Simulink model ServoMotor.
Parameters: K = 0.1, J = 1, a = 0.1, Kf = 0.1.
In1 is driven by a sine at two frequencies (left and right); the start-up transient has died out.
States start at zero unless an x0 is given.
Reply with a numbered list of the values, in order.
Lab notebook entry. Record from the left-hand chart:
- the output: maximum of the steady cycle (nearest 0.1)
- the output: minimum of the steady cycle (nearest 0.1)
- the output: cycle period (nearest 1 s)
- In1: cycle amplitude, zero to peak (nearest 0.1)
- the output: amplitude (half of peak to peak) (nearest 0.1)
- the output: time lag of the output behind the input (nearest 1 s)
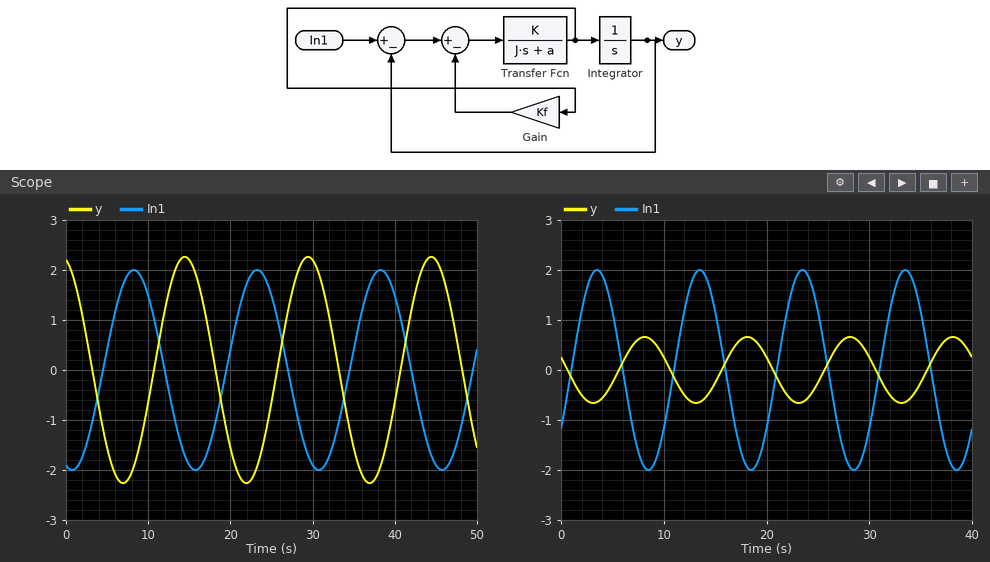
1. 2.3
2. -2.3
3. 15 s
4. 2.0
5. 2.3
6. 6 s
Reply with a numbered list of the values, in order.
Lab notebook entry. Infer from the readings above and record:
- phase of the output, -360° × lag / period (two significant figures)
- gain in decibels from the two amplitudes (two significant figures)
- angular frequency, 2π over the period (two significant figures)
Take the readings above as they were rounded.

1. -140°
2. 1.2 dB
3. 0.42 rad/s
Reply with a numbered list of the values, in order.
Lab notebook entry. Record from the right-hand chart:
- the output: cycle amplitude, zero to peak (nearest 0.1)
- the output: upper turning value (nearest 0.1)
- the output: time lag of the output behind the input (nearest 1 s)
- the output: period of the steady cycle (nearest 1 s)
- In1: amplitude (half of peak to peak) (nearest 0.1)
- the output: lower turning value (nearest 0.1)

1. 0.7
2. 0.7
3. 5 s
4. 10 s
5. 2.0
6. -0.7
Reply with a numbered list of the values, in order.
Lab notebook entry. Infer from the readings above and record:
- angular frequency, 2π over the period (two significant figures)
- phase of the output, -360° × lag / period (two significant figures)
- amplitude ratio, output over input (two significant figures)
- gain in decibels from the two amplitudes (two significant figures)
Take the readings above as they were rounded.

1. 0.63 rad/s
2. -180°
3. 0.35
4. -9.1 dB
